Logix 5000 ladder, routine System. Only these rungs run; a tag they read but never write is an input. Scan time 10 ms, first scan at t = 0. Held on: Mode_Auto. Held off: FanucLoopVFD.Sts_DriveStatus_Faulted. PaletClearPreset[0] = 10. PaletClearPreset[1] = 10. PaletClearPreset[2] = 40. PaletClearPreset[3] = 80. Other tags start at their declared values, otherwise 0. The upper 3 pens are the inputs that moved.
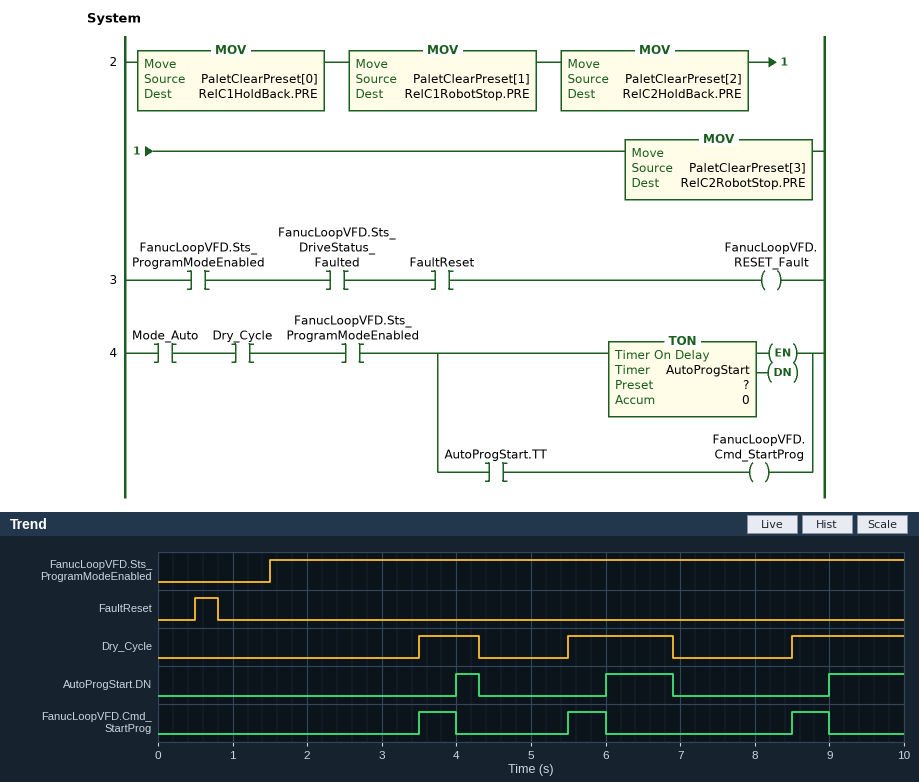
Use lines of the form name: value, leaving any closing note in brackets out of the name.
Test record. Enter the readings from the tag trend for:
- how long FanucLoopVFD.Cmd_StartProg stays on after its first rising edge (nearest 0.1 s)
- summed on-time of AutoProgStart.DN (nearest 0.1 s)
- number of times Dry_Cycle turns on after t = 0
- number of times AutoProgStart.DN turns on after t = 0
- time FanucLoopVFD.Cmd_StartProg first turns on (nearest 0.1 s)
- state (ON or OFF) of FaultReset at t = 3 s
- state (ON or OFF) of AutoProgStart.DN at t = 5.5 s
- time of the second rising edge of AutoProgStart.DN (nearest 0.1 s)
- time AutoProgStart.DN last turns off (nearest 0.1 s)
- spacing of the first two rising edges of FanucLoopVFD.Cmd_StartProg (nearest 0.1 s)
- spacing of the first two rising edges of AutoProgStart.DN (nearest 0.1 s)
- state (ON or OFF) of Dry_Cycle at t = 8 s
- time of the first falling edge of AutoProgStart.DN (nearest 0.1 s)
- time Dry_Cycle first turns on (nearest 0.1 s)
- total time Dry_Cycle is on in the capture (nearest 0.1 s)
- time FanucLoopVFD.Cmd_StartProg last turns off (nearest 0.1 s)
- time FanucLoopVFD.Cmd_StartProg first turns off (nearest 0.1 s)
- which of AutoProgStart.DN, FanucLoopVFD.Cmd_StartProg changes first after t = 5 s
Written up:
how long FanucLoopVFD.Cmd_StartProg stays on after its first rising edge: 0.5 s
summed on-time of AutoProgStart.DN: 2.2 s
number of times Dry_Cycle turns on after t = 0: 3
number of times AutoProgStart.DN turns on after t = 0: 3
time FanucLoopVFD.Cmd_StartProg first turns on: 3.5 s
state (ON or OFF) of FaultReset at t = 3 s: OFF
state (ON or OFF) of AutoProgStart.DN at t = 5.5 s: OFF
time of the second rising edge of AutoProgStart.DN: 6.0 s
time AutoProgStart.DN last turns off: 6.9 s
spacing of the first two rising edges of FanucLoopVFD.Cmd_StartProg: 2.0 s
spacing of the first two rising edges of AutoProgStart.DN: 2.0 s
state (ON or OFF) of Dry_Cycle at t = 8 s: OFF
time of the first falling edge of AutoProgStart.DN: 4.3 s
time Dry_Cycle first turns on: 3.5 s
total time Dry_Cycle is on in the capture: 3.7 s
time FanucLoopVFD.Cmd_StartProg last turns off: 9.0 s
time FanucLoopVFD.Cmd_StartProg first turns off: 4.0 s
which of AutoProgStart.DN, FanucLoopVFD.Cmd_StartProg changes first after t = 5 s: FanucLoopVFD.Cmd_StartProg
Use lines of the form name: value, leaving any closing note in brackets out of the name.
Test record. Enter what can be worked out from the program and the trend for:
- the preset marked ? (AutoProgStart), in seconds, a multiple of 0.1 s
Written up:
the preset marked ? (AutoProgStart), in seconds, a multiple of 0.1 s: 0.5 s
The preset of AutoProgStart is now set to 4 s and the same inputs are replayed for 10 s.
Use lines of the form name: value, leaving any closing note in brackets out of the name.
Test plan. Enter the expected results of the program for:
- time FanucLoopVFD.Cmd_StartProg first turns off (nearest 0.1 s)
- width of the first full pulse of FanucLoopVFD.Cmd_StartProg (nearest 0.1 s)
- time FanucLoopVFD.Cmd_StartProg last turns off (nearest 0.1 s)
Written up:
time FanucLoopVFD.Cmd_StartProg first turns off: 4.3 s
width of the first full pulse of FanucLoopVFD.Cmd_StartProg: 0.8 s
time FanucLoopVFD.Cmd_StartProg last turns off: 6.9 s
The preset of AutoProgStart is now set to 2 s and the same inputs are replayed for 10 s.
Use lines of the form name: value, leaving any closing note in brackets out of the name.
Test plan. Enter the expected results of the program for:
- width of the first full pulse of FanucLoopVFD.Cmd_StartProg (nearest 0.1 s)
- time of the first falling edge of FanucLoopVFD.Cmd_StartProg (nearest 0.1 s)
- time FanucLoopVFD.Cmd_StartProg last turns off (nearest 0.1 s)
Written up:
width of the first full pulse of FanucLoopVFD.Cmd_StartProg: 0.8 s
time of the first falling edge of FanucLoopVFD.Cmd_StartProg: 4.3 s
time FanucLoopVFD.Cmd_StartProg last turns off: 6.9 s
